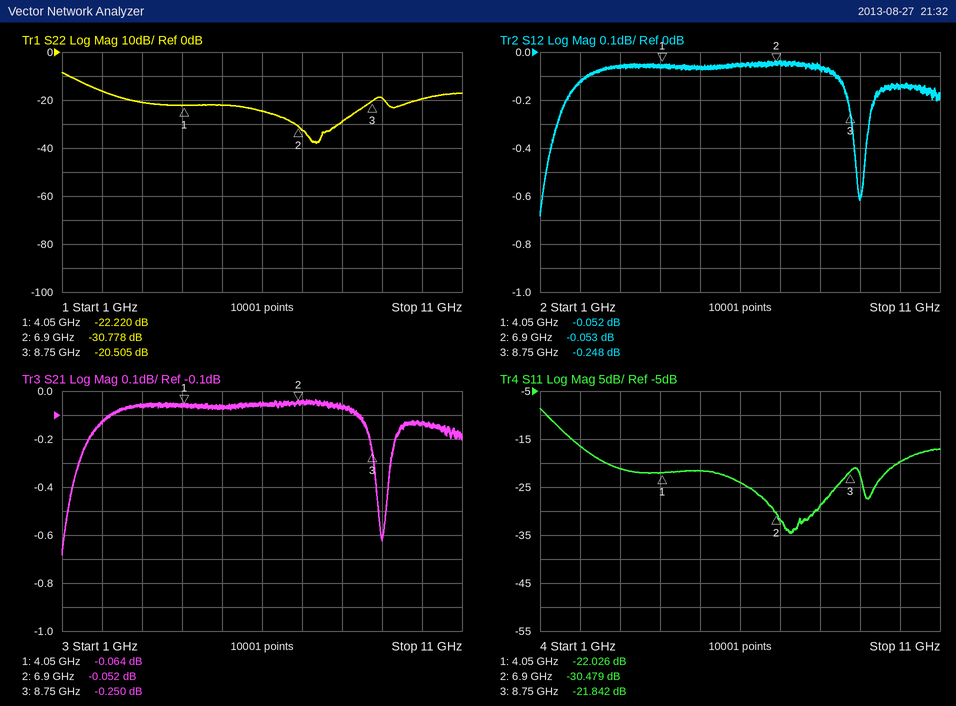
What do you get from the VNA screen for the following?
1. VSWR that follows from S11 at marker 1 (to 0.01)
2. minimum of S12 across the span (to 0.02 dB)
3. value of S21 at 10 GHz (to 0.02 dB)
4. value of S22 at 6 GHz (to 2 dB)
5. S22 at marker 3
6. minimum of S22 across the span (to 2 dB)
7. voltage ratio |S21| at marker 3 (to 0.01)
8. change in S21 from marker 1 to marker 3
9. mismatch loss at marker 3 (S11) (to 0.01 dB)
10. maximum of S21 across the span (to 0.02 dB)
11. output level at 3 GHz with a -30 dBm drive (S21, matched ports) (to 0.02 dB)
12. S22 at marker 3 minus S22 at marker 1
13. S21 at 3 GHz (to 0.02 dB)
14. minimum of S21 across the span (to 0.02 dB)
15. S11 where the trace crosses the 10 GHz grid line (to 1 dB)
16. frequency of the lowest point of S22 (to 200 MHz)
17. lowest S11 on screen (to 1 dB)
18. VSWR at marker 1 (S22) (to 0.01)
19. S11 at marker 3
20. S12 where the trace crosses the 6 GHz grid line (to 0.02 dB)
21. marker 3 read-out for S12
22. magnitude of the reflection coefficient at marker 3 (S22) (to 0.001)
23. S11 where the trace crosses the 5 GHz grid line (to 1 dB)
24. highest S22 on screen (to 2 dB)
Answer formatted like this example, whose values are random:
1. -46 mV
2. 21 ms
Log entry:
1. 1.17
2. -0.68 dB
3. -0.14 dB
4. -24 dB
5. -20.505 dB
6. -38 dB
7. 0.97
8. -0.186 dB
9. 0.03 dB
10. -0.04 dB
11. -30.06 dBm
12. 1.715 dB
13. -0.06 dB
14. -0.68 dB
15. -20 dB
16. 7.4 GHz
17. -35 dB
18. 1.17
19. -21.842 dB
20. -0.06 dB
21. -0.248 dB
22. 0.094
23. -22 dB
24. -8 dB
